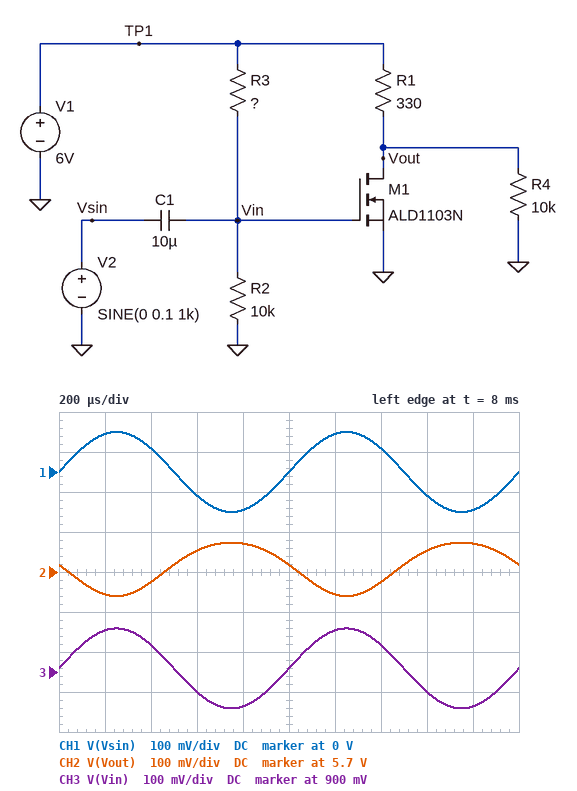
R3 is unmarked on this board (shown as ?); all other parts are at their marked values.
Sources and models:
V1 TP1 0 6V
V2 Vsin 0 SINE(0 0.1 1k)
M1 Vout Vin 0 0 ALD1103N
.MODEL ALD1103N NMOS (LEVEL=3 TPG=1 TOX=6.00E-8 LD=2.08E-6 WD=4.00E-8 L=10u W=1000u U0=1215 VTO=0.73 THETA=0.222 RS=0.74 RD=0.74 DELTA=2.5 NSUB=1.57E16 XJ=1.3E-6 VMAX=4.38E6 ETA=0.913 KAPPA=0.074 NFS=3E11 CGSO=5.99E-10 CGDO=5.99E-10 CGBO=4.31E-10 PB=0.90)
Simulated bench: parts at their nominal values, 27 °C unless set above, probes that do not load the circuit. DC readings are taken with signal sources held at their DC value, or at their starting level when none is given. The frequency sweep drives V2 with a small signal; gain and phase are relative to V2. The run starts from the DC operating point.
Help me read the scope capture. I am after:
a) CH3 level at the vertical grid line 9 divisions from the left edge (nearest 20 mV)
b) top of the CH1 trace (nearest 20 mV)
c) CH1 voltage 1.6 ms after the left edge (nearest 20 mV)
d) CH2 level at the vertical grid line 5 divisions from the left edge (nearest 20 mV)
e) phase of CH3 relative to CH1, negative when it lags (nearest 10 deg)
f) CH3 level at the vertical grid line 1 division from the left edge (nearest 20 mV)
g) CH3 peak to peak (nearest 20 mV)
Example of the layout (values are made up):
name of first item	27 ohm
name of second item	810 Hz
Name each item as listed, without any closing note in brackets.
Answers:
CH3 level at the vertical grid line 9 divisions from the left edge	820 mV
top of the CH1 trace	100 mV
CH1 voltage 1.6 ms after the left edge	-60 mV
CH2 level at the vertical grid line 5 divisions from the left edge	5.72 V
phase of CH3 relative to CH1, negative when it lags	0 deg
CH3 level at the vertical grid line 1 division from the left edge	1.00 V
CH3 peak to peak	200 mV
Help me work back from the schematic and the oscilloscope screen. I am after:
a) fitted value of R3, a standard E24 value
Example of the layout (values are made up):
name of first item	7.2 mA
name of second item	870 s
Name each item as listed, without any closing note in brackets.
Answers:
fitted value of R3, a standard E24 value	56 kΩ
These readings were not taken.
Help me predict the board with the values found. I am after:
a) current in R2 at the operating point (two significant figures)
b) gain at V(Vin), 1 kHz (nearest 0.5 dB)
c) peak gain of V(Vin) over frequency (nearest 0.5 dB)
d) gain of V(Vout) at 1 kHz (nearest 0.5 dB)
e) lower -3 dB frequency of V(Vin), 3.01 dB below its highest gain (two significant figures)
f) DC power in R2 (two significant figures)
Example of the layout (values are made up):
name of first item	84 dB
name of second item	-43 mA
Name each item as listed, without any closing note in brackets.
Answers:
current in R2 at the operating point	91 µA
gain at V(Vin), 1 kHz	0 dB
peak gain of V(Vin) over frequency	0 dB
gain of V(Vout) at 1 kHz	-3.5 dB
lower -3 dB frequency of V(Vin), 3.01 dB below its highest gain	1.9 Hz
DC power in R2	83 µW
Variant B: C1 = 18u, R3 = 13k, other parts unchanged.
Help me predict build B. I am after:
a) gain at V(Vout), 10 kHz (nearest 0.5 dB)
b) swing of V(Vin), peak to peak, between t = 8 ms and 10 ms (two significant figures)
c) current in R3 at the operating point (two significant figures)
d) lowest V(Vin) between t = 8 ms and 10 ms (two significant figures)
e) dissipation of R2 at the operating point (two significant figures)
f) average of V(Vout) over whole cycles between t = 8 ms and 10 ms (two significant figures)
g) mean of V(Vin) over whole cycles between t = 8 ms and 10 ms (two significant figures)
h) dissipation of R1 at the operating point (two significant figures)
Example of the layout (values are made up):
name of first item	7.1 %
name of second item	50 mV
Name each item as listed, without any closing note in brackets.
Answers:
gain at V(Vout), 10 kHz	10.0 dB
swing of V(Vin), peak to peak, between t = 8 ms and 10 ms	200 mV
current in R3 at the operating point	260 µA
lowest V(Vin) between t = 8 ms and 10 ms	2.5 V
dissipation of R2 at the operating point	680 µW
average of V(Vout) over whole cycles between t = 8 ms and 10 ms	2.2 V
mean of V(Vin) over whole cycles between t = 8 ms and 10 ms	2.6 V
dissipation of R1 at the operating point	45 mW
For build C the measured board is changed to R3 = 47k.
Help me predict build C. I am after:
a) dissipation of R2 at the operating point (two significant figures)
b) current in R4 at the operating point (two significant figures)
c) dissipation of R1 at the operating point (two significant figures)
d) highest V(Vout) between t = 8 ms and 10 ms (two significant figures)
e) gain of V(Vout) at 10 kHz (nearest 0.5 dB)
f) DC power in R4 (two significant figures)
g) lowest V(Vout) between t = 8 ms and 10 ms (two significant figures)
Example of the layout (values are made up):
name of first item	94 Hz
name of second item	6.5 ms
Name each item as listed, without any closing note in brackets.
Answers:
dissipation of R2 at the operating point	110 µW
current in R4 at the operating point	560 µA
dissipation of R1 at the operating point	490 µW
highest V(Vout) between t = 8 ms and 10 ms	5.7 V
gain of V(Vout) at 10 kHz	0 dB
DC power in R4	3.1 mW
lowest V(Vout) between t = 8 ms and 10 ms	5.5 V
